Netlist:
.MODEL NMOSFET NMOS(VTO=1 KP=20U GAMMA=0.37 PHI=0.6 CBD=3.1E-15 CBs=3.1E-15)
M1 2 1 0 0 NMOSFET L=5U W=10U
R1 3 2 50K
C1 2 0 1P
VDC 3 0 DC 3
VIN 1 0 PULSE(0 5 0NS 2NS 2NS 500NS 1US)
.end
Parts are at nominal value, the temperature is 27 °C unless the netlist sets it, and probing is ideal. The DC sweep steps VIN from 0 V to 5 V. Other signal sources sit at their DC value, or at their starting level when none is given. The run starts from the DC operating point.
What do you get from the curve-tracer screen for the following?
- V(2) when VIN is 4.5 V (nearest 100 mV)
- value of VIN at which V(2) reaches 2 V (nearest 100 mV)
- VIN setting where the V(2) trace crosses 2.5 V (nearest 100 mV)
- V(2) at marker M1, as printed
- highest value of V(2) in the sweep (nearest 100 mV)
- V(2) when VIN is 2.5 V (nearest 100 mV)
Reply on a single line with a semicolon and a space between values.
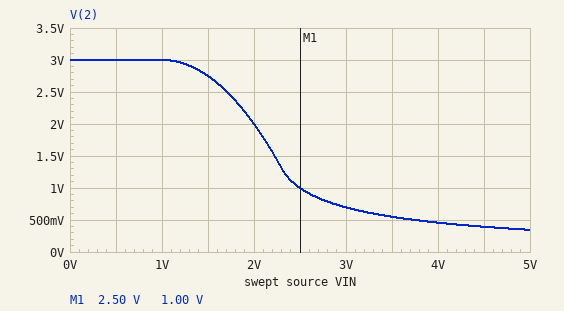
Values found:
400 mV; 2.0 V; 1.7 V; 1.00 V; 3.0 V; 1.0 V
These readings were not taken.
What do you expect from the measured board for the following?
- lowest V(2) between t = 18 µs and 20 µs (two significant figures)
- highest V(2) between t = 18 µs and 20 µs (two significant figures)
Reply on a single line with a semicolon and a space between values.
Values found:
350 mV; 3.0 V
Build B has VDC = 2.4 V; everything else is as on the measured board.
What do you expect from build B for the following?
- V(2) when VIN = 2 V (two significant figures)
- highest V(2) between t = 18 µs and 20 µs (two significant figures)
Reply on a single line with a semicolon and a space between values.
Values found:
1.4 V; 2.4 V
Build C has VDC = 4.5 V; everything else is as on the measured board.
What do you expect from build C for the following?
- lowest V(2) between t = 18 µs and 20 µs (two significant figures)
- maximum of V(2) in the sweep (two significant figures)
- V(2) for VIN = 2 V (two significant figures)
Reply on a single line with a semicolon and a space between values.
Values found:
530 mV; 4.5 V; 3.5 V
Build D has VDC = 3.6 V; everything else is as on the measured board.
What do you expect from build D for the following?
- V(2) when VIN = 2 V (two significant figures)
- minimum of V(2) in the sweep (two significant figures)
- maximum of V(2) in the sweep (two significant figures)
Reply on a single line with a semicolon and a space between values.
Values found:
2.6 V; 420 mV; 3.6 V
